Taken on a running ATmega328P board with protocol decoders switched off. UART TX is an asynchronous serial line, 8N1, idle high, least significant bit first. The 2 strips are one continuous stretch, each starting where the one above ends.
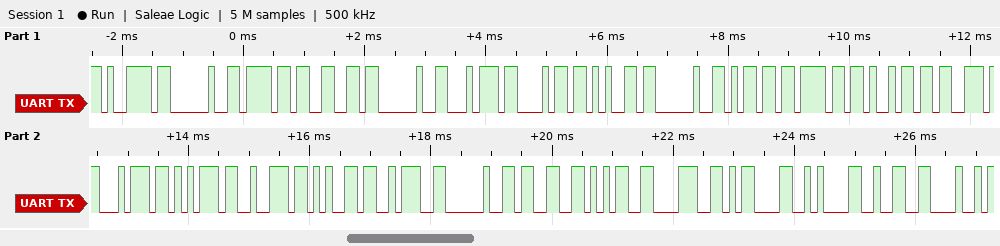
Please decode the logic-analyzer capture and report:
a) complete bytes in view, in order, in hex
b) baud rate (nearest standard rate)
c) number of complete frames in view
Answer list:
79 20 6F 66 20 74 68 65 20 6D 6F 69 73 74 75 72 65 3A 20 33 35 38 0D 0A 32 48
9600 baud
26
